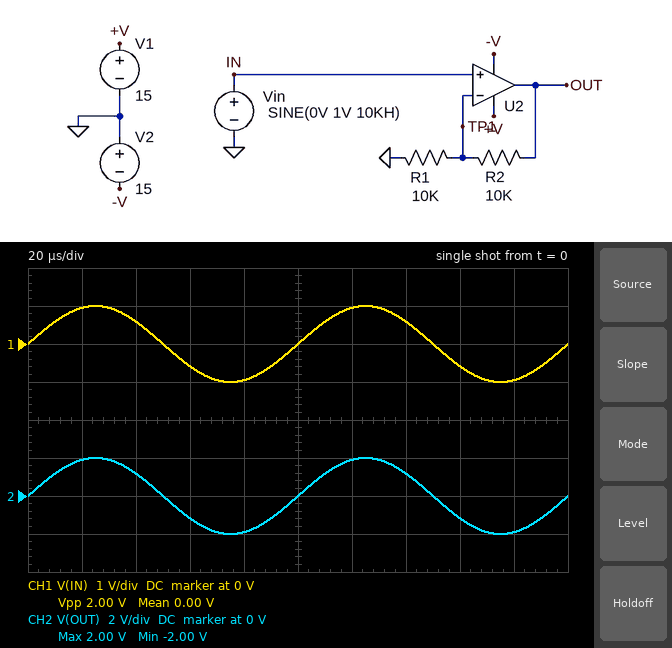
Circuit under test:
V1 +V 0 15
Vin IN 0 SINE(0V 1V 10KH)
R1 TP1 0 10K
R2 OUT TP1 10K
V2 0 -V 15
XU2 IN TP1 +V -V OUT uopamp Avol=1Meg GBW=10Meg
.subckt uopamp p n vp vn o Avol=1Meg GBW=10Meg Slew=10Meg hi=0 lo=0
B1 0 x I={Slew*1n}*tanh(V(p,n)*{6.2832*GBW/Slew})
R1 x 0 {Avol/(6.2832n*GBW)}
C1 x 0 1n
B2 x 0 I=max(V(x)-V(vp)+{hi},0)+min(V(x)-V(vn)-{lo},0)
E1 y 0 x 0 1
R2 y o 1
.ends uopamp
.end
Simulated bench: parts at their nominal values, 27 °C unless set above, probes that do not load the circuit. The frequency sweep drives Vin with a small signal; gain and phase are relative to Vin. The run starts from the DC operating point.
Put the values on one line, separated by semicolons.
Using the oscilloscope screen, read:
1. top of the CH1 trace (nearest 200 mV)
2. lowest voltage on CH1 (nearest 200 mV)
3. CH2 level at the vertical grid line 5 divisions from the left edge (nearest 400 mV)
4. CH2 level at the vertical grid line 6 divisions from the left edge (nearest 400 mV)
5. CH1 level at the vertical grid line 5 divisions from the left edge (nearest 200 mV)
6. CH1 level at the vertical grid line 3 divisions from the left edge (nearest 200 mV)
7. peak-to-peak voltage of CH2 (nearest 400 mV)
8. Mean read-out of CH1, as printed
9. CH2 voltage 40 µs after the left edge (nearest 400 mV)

1.0 V; -1.0 V; 0 V; 2.0 V; 0 V; -600 mV; 4.0 V; 0.00 V; 1.2 V
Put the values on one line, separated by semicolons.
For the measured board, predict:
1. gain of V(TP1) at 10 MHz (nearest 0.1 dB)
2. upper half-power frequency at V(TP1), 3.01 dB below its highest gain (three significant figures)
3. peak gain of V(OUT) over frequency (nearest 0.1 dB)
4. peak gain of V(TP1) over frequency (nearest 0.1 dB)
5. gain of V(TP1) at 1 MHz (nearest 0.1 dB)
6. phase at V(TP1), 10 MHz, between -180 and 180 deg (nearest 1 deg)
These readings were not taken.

-7.0 dB; 5.00 MHz; 6.0 dB; 0 dB; -0.2 dB; -63 deg
